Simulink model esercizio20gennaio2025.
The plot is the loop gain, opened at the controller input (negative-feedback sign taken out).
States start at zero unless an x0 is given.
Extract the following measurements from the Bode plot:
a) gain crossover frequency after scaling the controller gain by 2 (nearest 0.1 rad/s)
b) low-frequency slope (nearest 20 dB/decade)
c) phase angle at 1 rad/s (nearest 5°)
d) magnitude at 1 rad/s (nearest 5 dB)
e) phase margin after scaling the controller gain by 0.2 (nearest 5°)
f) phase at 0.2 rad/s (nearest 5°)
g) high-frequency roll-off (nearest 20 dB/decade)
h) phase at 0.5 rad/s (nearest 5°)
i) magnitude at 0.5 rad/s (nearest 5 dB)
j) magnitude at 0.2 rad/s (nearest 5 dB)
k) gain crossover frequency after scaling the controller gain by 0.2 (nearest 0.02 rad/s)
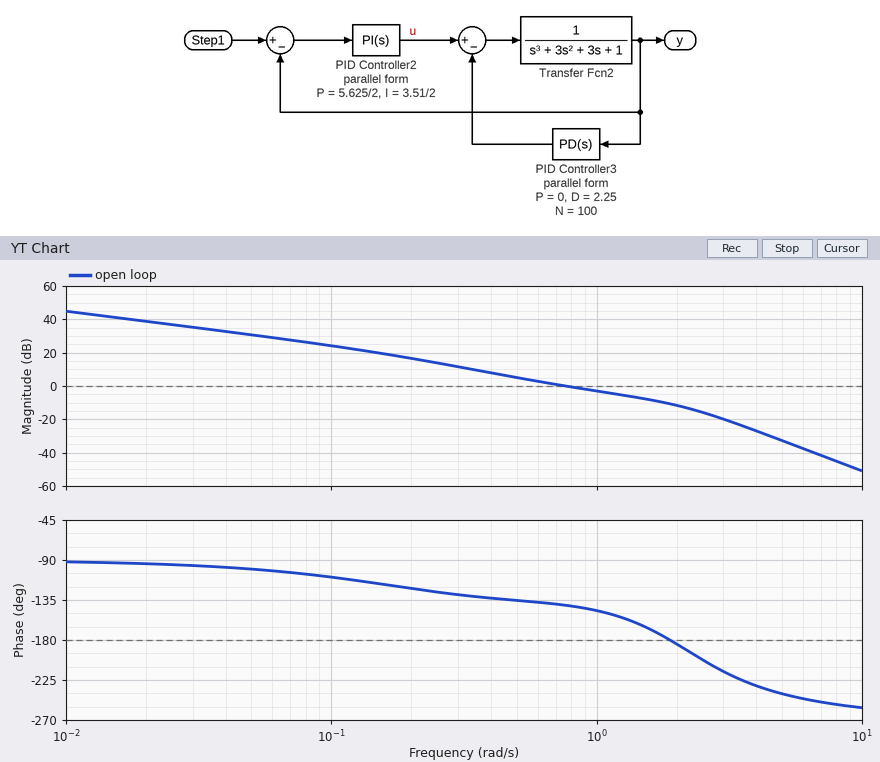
1.3 rad/s
-20 dB/decade
-145°
-5 dB
55°
-120°
-60 dB/decade
-135°
5 dB
15 dB
0.24 rad/s
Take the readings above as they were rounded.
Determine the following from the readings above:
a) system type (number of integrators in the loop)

1
